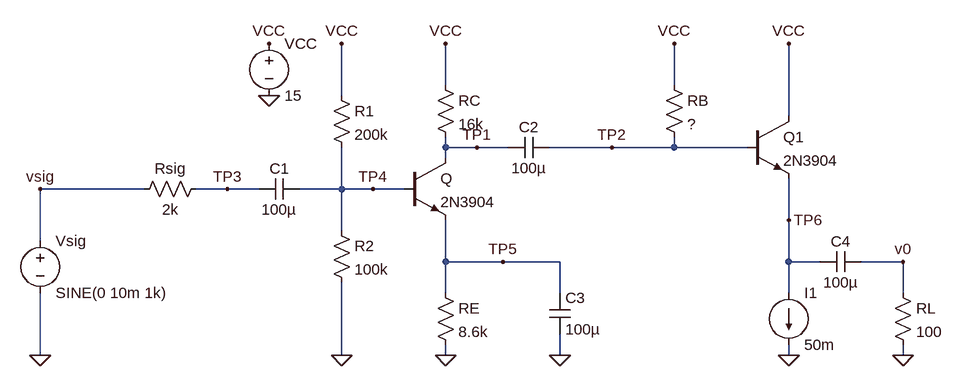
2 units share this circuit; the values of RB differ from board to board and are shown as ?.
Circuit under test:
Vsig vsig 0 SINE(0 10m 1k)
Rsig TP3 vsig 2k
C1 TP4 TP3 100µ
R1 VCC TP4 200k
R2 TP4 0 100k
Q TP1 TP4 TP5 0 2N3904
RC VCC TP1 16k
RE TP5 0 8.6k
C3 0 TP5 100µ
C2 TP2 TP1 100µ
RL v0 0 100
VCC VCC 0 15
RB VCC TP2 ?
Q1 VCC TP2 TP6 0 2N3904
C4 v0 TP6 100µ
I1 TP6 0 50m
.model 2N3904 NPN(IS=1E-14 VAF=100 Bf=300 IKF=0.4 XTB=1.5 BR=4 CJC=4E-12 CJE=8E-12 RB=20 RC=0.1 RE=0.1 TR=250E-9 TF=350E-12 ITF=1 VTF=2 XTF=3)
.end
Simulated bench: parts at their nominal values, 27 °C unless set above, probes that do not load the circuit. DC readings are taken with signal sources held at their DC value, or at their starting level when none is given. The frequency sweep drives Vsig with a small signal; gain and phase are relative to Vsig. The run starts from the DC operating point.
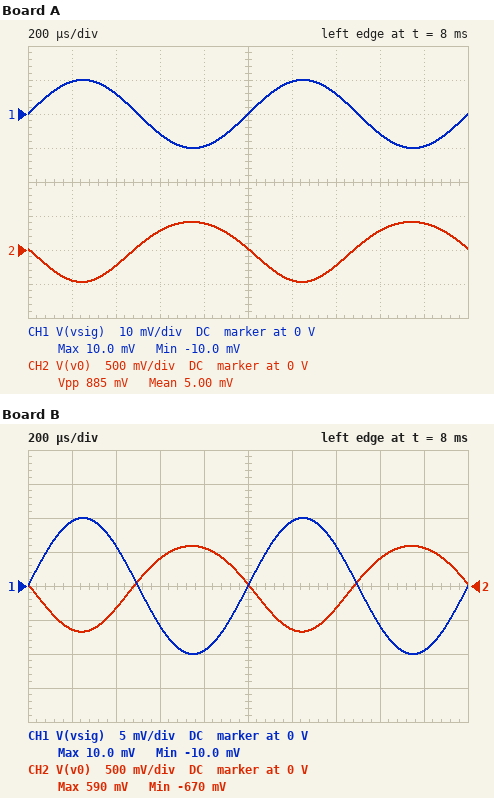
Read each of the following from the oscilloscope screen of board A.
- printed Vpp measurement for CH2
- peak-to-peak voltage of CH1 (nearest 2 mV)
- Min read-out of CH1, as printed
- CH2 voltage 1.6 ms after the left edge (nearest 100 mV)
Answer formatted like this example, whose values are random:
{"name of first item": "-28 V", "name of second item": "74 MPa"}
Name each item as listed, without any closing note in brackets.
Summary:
{"printed Vpp measurement for CH2": "885 mV", "peak-to-peak voltage of CH1": "20 mV", "Min read-out of CH1, as printed": "-10.0 mV", "CH2 voltage 1.6 ms after the left edge": "300 mV"}
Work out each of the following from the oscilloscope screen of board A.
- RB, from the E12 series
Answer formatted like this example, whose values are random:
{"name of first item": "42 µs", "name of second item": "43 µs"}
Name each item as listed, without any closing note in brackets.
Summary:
{"RB, from the E12 series": "3.9 kΩ"}
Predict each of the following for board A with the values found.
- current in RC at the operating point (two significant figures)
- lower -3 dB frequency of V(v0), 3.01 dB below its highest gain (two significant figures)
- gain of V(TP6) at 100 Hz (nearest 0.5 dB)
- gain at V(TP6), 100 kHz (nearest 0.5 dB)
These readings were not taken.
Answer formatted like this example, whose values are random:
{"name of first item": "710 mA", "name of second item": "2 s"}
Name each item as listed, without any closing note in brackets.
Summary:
{"current in RC at the operating point": "490 µA", "lower -3 dB frequency of V(v0), 3.01 dB below its highest gain": "33 Hz", "gain of V(TP6) at 100 Hz": "32.5 dB", "gain at V(TP6), 100 kHz": "33.0 dB"}
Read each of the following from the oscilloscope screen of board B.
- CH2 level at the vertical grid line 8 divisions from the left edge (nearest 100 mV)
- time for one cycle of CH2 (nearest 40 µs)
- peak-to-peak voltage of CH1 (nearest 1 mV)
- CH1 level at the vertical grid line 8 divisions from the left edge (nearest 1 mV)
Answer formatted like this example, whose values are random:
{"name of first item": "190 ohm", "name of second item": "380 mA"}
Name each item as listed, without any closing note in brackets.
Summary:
{"CH2 level at the vertical grid line 8 divisions from the left edge": "400 mV", "time for one cycle of CH2": "1.00 ms", "peak-to-peak voltage of CH1": "20 mV", "CH1 level at the vertical grid line 8 divisions from the left edge": "-6 mV"}
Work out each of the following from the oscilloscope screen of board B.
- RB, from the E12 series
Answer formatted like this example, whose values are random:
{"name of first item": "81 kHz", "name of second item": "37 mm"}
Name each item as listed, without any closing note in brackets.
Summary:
{"RB, from the E12 series": "6.8 kΩ"}
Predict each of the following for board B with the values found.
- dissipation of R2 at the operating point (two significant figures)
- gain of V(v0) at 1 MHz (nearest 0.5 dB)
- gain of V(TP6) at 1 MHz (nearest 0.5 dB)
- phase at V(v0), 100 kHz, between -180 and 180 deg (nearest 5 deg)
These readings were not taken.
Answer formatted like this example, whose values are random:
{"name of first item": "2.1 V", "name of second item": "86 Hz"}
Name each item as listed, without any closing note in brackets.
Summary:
{"dissipation of R2 at the operating point": "240 µW", "gain of V(v0) at 1 MHz": "27.5 dB", "gain of V(TP6) at 1 MHz": "27.5 dB", "phase at V(v0), 100 kHz, between -180 and 180 deg": "165 deg"}
